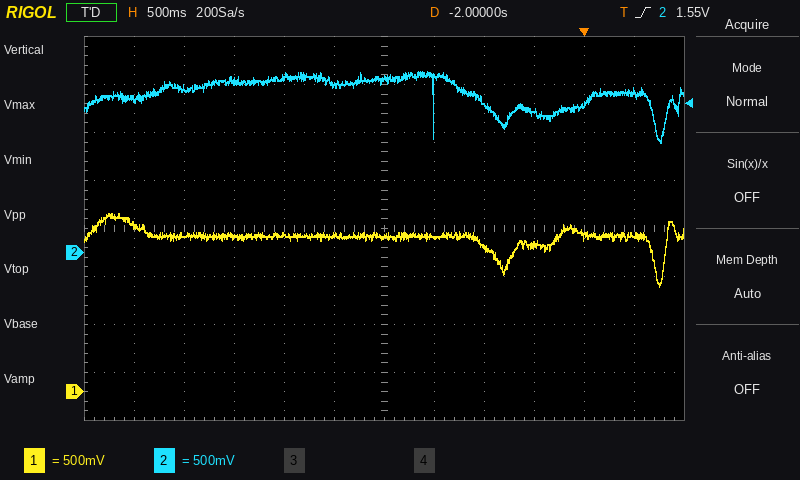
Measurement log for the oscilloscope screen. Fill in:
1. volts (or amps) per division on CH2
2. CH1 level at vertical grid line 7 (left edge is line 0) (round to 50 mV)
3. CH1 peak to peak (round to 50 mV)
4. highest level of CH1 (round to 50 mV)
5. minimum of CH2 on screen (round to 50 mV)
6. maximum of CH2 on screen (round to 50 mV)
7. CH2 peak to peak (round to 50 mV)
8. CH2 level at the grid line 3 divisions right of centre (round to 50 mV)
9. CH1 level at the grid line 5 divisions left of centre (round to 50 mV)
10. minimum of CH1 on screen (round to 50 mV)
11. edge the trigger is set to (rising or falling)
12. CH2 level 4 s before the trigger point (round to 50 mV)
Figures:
500 mV
1.60 V
750 mV
1.85 V
1.15 V
1.90 V
750 mV
1.45 V
1.75 V
1.10 V
rising
1.70 V
